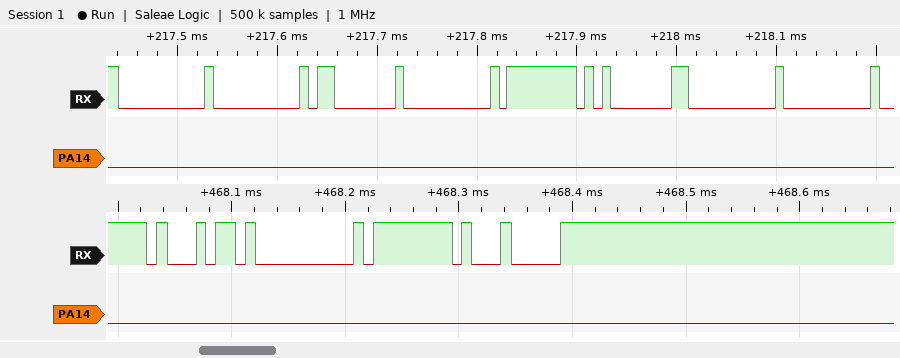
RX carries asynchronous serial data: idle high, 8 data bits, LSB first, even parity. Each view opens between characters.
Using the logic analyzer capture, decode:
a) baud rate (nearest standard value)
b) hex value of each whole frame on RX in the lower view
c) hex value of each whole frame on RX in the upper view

115200 baud
D1, 00, FF, 04
00, 00, 03, 00, FF, 01, 00, 00
